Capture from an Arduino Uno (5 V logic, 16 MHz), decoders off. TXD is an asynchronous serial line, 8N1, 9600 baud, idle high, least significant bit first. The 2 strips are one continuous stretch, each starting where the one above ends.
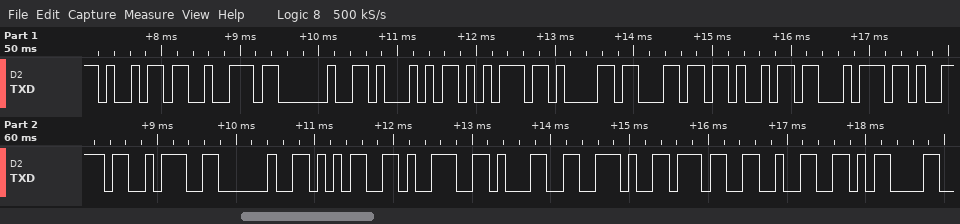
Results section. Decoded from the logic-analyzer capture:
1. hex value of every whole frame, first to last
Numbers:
0x69 0x72 0x20 0x51 0x75 0x61 0x6C 0x69 0x74 0x79 0x3A 0x20 0x35 0x39 0x31 0x2E 0x37 0x32 0x0D
